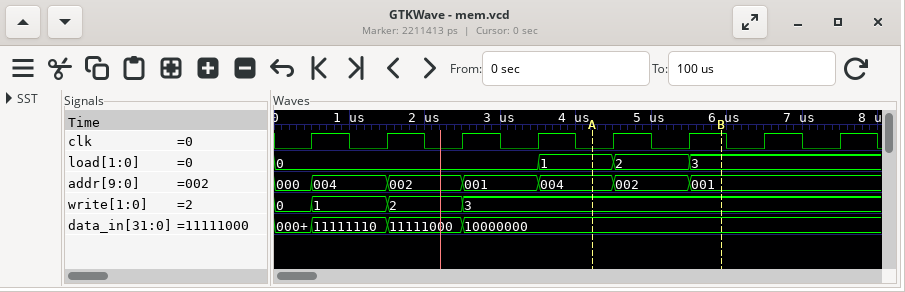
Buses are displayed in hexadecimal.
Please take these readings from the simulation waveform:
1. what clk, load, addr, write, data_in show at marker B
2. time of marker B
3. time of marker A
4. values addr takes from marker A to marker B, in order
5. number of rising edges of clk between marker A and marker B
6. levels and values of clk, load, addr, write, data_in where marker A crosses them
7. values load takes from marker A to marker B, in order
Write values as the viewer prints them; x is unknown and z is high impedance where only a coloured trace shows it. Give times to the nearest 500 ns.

clk=1, load=3, addr=001, write=3, data_in=10000000
6000 ns
4000 ns
004, 002, 001
2
clk=0, load=1, addr=004, write=3, data_in=10000000
1, 2, 3
